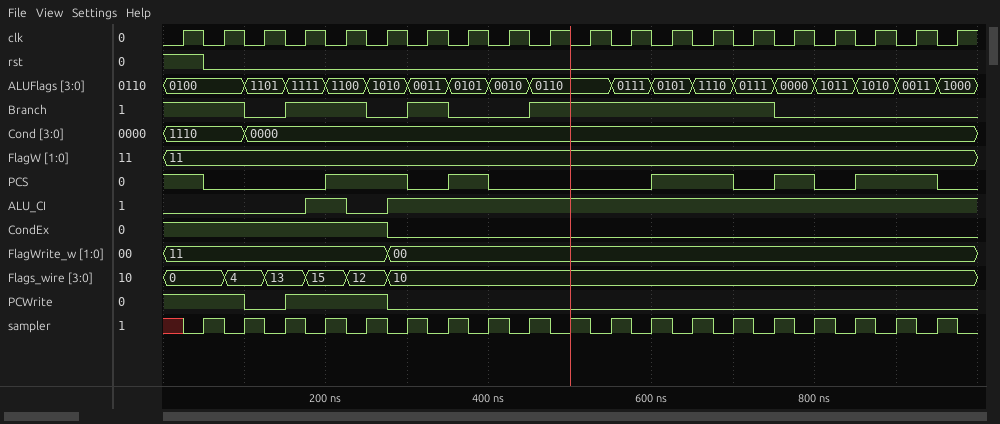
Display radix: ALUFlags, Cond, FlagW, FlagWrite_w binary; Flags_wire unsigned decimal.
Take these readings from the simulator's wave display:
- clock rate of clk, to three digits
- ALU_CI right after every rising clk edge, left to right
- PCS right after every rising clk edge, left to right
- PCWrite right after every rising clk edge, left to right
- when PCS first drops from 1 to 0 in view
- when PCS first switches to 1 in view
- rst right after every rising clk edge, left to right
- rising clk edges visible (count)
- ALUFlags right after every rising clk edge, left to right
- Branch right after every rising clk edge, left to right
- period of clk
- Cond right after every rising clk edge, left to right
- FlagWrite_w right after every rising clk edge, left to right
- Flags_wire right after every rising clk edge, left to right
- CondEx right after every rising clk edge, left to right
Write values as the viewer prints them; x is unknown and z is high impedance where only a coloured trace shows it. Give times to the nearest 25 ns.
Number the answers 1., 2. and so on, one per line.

1. 20.0 MHz
2. 0 0 0 1 0 1 1 1 1 1 1 1 1 1 1 1 1 1 1 1
3. 1 0 0 0 1 1 0 1 0 0 0 0 1 1 0 1 0 1 1 0
4. 1 1 0 1 1 0 0 0 0 0 0 0 0 0 0 0 0 0 0 0
5. 50 ns
6. 200 ns
7. 1 0 0 0 0 0 0 0 0 0 0 0 0 0 0 0 0 0 0 0
8. 20
9. 0100, 0100, 1101, 1111, 1100, 1010, 0011, 0101, 0010, 0110, 0110, 0111, 0101, 1110, 0111, 0000, 1011, 1010, 0011, 1000
10. 1 1 0 1 1 0 1 0 0 1 1 1 1 1 1 0 0 0 0 0
11. 50 ns
12. 1110, 1110, 0000, 0000, 0000, 0000, 0000, 0000, 0000, 0000, 0000, 0000, 0000, 0000, 0000, 0000, 0000, 0000, 0000, 0000
13. 11, 11, 11, 11, 11, 00, 00, 00, 00, 00, 00, 00, 00, 00, 00, 00, 00, 00, 00, 00
14. 0, 4, 13, 15, 12, 10, 10, 10, 10, 10, 10, 10, 10, 10, 10, 10, 10, 10, 10, 10
15. 1 1 1 1 1 0 0 0 0 0 0 0 0 0 0 0 0 0 0 0
